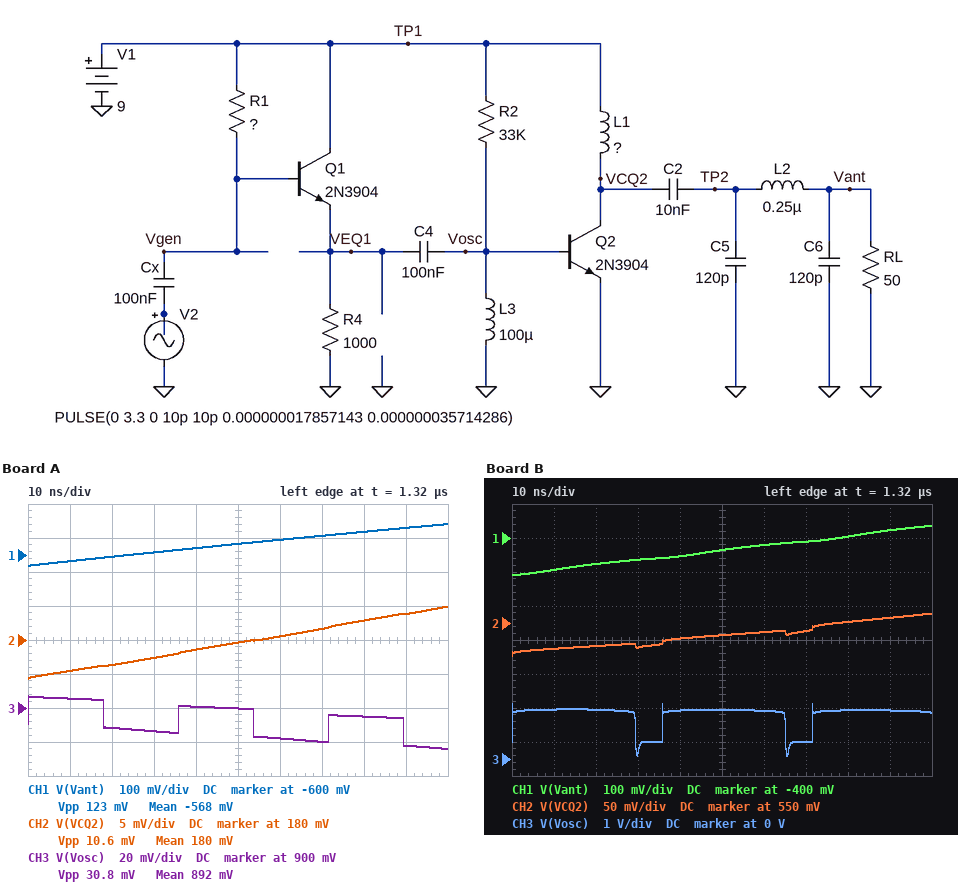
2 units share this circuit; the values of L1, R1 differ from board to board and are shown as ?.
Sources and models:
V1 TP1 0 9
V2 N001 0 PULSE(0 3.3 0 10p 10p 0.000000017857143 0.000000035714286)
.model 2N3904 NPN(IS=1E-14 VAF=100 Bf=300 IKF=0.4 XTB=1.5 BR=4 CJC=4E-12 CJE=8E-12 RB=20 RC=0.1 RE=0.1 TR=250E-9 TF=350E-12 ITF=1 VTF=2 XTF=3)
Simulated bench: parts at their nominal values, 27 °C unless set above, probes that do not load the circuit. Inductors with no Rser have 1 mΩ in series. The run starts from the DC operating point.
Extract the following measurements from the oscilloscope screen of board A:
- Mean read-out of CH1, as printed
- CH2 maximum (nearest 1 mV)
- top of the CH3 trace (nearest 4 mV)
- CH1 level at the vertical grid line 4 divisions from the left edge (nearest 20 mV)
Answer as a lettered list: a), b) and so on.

a) -568 mV
b) 185 mV
c) 908 mV
d) -580 mV
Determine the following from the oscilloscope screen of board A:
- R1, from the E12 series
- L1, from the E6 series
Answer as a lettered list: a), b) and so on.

a) 15 kΩ
b) 33 µH
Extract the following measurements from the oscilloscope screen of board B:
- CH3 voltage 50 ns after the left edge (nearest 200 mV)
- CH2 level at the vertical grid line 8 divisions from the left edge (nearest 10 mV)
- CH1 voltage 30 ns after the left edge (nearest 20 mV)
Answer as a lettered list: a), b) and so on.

a) 1.4 V
b) 550 mV
c) -460 mV
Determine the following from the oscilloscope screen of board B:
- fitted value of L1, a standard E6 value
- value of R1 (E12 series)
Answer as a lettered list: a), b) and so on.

a) 6.8 µH
b) 56 kΩ
